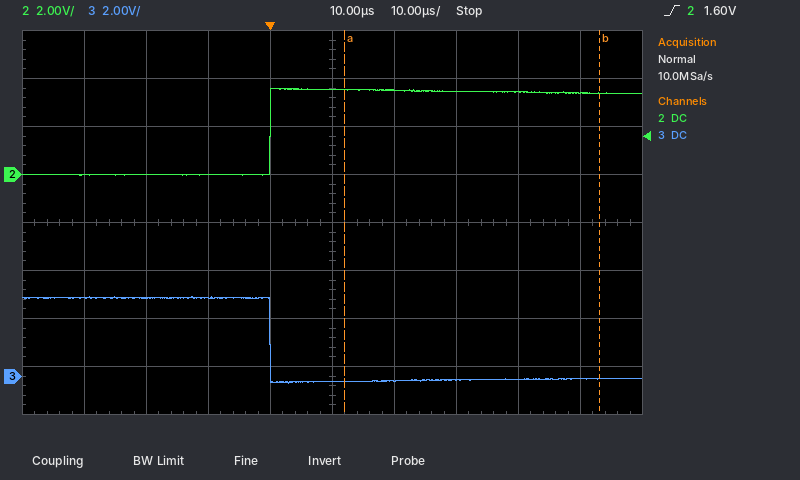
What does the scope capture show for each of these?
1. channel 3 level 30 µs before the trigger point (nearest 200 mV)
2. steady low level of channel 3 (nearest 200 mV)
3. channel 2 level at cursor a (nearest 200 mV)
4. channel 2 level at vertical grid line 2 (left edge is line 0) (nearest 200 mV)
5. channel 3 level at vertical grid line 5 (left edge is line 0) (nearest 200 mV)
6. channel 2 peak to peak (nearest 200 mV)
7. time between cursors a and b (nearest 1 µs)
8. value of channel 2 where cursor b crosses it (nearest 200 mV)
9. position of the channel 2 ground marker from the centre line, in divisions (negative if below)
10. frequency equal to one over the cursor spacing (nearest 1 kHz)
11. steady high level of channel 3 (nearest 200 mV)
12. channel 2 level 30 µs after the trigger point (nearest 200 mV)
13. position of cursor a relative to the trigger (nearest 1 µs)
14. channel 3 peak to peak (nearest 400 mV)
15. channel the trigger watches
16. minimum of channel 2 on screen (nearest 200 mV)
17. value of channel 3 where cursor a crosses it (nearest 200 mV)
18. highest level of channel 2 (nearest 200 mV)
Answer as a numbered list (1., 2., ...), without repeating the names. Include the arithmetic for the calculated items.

1. 3.2 V
2. -200 mV
3. 3.6 V
4. 0.0 V
5. -200 mV
6. 3.6 V − (0.0 V) = 3.6 V
7. 41 µs
8. 3.4 V
9. +1.0 div
10. 1 / 41 µs ≈ 24 kHz
11. 3.2 V
12. 3.4 V
13. +12 µs
14. 3.6 V
15. channel 2
16. 0.0 V
17. -200 mV
18. 3.6 V
